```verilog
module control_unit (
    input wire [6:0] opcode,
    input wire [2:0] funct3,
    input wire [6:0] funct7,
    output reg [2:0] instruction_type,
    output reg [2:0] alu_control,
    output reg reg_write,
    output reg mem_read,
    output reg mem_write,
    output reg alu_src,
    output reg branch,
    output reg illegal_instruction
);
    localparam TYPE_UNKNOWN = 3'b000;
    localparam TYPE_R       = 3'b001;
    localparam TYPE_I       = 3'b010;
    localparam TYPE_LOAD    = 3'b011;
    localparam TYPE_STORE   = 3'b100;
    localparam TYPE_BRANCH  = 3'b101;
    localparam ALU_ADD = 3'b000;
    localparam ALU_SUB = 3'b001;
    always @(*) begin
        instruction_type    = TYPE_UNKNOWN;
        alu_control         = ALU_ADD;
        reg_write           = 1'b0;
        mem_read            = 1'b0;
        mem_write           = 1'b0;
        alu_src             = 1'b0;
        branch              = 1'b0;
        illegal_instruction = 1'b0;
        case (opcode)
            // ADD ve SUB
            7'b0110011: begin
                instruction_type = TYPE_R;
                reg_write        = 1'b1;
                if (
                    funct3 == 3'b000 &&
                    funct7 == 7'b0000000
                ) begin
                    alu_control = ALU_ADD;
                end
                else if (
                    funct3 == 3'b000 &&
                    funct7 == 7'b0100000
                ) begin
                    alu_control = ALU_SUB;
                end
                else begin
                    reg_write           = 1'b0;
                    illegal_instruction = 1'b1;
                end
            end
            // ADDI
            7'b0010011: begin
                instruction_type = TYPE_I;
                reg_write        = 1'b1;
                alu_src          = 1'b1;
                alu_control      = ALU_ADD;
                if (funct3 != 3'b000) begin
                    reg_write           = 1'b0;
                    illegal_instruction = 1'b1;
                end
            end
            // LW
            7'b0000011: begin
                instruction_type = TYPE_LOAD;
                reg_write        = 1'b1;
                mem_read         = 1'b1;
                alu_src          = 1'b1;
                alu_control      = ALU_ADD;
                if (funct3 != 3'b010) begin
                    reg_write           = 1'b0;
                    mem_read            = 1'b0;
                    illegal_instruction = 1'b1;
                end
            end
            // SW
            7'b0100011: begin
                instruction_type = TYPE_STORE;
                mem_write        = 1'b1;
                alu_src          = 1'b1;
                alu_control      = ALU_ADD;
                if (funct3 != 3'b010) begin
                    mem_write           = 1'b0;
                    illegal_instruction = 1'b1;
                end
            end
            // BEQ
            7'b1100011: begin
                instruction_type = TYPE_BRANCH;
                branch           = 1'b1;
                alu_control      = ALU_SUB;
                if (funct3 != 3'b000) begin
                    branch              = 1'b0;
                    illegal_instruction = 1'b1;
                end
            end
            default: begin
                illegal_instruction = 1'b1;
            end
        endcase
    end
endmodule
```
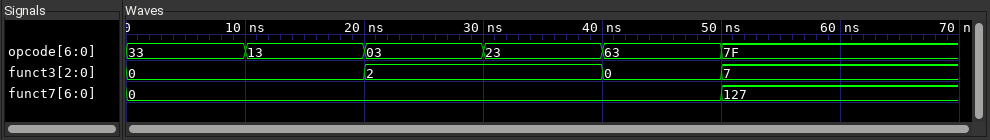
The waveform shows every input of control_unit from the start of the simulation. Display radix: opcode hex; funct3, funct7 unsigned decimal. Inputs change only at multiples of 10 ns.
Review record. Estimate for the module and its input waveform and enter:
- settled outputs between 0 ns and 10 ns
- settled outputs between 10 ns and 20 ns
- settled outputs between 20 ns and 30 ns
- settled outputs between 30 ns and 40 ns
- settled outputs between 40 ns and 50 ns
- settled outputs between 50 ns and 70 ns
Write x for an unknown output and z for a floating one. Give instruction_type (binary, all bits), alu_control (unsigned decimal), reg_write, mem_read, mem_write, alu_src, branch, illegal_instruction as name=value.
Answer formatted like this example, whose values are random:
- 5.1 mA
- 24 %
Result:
- instruction_type=001, alu_control=0, reg_write=1, mem_read=0, mem_write=0, alu_src=0, branch=0, illegal_instruction=0
- instruction_type=010, alu_control=0, reg_write=1, mem_read=0, mem_write=0, alu_src=1, branch=0, illegal_instruction=0
- instruction_type=011, alu_control=0, reg_write=1, mem_read=1, mem_write=0, alu_src=1, branch=0, illegal_instruction=0
- instruction_type=100, alu_control=0, reg_write=0, mem_read=0, mem_write=1, alu_src=1, branch=0, illegal_instruction=0
- instruction_type=101, alu_control=1, reg_write=0, mem_read=0, mem_write=0, alu_src=0, branch=1, illegal_instruction=0
- instruction_type=000, alu_control=0, reg_write=0, mem_read=0, mem_write=0, alu_src=0, branch=0, illegal_instruction=1
